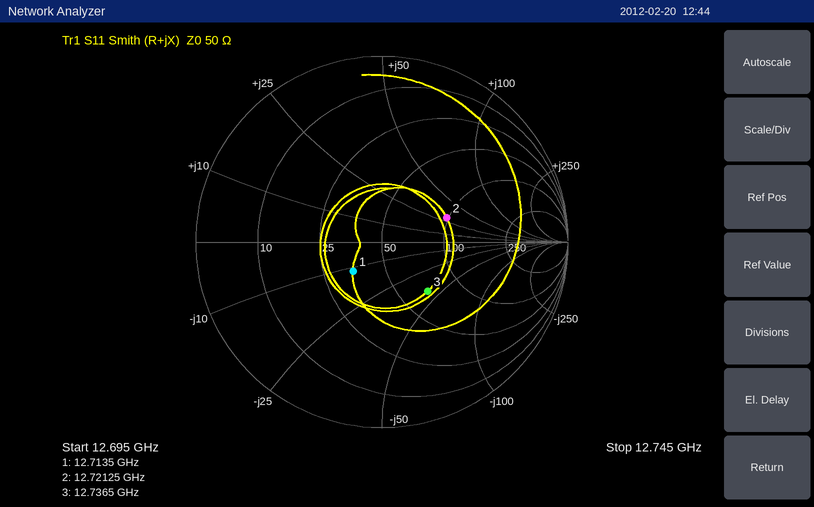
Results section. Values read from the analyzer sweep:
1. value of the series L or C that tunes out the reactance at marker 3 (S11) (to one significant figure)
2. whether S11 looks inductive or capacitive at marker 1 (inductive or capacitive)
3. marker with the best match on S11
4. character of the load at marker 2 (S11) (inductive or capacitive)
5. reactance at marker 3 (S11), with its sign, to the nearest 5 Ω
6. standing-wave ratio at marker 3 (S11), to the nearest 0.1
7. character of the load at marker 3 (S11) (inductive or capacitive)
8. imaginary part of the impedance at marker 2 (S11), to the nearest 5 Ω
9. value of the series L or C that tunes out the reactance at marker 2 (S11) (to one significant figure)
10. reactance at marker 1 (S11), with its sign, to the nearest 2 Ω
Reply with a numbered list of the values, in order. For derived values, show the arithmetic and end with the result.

1. L = 40 Ω/(2π × 12.7365 GHz) ≈ 500 pH
2. capacitive
3. marker 1
4. inductive
5. -40 Ω
6. 2.1
7. capacitive
8. +30 Ω
9. C = 1/(2π × 12.72125 GHz × 30 Ω) ≈ 417 fF, so 400 fF to one significant figure
10. -12 Ω
